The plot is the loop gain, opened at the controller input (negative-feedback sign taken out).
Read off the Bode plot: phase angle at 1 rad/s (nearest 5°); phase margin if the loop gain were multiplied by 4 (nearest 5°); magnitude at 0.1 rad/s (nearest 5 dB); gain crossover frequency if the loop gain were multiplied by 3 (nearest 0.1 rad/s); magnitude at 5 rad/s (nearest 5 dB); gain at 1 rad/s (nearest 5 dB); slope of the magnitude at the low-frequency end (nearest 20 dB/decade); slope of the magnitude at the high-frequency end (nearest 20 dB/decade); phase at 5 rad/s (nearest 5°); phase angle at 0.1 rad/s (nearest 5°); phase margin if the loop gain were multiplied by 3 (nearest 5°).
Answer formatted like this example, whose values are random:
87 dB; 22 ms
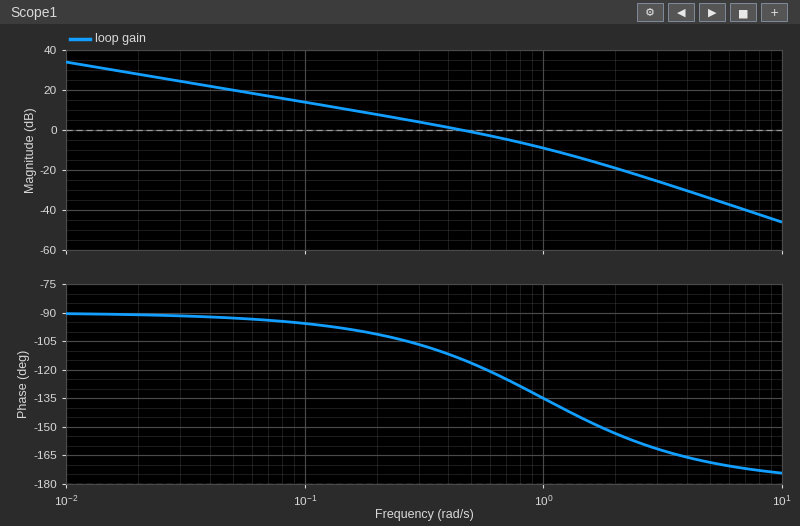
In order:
-135°; 40°; 15 dB; 1.0 rad/s; -35 dB; -10 dB; -20 dB/decade; -40 dB/decade; -170°; -95°; 45°
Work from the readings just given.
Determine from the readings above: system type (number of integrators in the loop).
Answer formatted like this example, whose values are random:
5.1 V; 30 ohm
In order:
1
